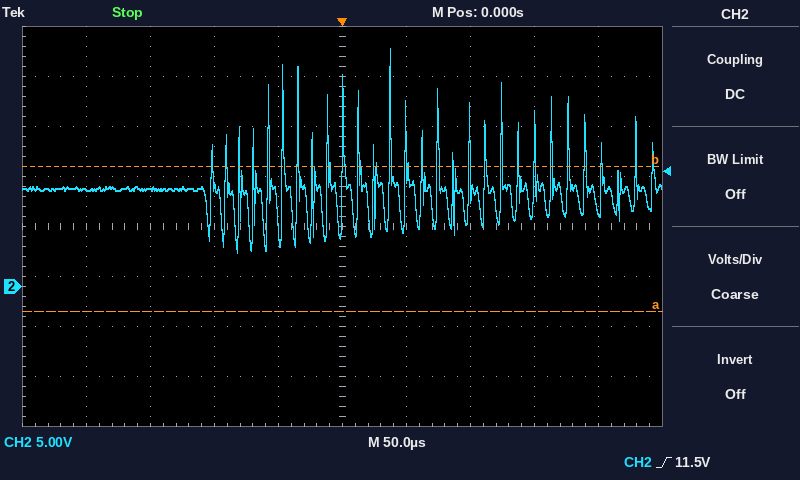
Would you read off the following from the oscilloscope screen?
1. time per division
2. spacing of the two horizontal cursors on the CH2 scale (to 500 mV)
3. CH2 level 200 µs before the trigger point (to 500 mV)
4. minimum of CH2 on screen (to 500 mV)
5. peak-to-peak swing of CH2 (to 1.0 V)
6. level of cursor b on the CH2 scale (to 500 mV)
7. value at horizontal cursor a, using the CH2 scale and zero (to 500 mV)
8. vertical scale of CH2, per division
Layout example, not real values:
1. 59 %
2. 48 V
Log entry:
1. 50 µs
2. 14.5 V
3. 9.5 V
4. 3.5 V
5. 20.0 V
6. 12.0 V
7. -2.5 V
8. 5 V
